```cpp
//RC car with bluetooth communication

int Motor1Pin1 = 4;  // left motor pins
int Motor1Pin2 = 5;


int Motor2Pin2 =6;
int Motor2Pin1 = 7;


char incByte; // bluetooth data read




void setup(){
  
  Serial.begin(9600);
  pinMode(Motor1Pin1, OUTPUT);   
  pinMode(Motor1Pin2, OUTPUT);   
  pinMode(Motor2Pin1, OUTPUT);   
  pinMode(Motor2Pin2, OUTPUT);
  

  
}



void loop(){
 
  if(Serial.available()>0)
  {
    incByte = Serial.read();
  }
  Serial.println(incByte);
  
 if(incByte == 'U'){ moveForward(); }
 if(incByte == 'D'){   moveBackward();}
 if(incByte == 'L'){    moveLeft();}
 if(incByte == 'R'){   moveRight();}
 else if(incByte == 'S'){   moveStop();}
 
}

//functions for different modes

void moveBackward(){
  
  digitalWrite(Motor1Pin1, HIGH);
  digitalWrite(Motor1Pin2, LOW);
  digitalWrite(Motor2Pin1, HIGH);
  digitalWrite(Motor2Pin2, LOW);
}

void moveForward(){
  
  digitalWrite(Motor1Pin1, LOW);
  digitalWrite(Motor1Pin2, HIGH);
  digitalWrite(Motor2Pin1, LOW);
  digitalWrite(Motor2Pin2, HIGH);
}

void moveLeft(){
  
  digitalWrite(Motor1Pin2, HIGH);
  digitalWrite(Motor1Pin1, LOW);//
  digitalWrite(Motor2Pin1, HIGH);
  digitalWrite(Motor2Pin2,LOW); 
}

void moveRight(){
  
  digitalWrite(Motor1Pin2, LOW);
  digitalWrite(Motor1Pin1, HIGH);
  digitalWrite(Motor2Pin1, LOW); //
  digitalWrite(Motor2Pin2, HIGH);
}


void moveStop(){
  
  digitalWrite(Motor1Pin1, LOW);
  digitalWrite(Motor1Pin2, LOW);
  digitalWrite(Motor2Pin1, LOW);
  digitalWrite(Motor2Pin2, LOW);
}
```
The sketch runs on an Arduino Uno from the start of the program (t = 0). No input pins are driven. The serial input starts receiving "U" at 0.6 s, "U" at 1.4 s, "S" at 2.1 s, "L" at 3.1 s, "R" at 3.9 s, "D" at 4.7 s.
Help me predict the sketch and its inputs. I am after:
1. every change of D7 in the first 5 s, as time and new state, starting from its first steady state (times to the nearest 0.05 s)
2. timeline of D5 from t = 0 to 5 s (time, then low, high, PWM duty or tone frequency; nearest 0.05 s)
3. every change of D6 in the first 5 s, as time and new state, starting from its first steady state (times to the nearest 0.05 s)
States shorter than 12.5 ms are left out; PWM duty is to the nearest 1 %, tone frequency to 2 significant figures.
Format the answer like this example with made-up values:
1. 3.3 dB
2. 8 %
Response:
1. 0 s low; 3.1 s high; 3.9 s low; 4.7 s high
2. 0 s low; 0.6 s high; 2.1 s low; 3.1 s high; 3.9 s low
3. 0 s low; 0.6 s high; 2.1 s low; 3.9 s high; 4.7 s low
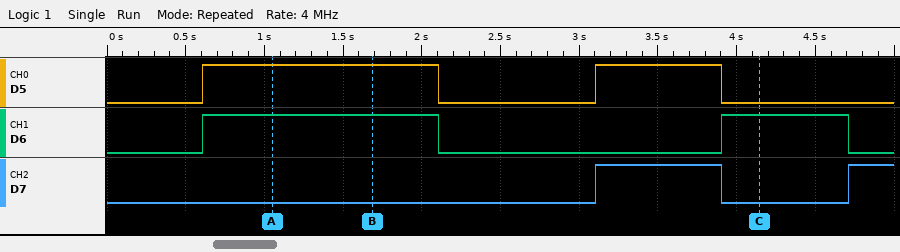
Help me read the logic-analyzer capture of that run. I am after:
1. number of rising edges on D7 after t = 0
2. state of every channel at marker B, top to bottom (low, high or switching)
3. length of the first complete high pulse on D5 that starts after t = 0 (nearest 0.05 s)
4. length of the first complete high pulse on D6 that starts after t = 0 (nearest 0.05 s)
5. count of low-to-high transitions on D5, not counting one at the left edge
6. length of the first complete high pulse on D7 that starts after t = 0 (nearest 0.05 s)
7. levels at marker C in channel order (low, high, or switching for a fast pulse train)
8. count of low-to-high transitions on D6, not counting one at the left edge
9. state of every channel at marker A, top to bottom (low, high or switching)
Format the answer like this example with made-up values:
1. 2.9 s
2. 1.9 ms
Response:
1. 2
2. D5 high, D6 high, D7 low
3. 1.50 s
4. 1.50 s
5. 2
6. 0.80 s
7. D5 low, D6 high, D7 low
8. 2
9. D5 high, D6 high, D7 low
